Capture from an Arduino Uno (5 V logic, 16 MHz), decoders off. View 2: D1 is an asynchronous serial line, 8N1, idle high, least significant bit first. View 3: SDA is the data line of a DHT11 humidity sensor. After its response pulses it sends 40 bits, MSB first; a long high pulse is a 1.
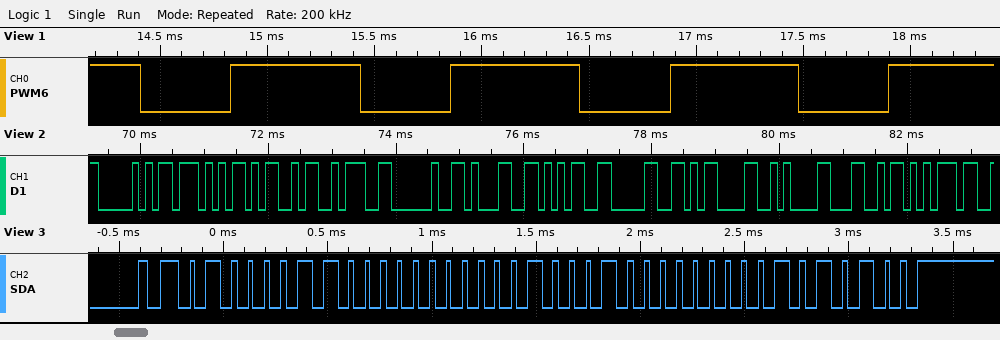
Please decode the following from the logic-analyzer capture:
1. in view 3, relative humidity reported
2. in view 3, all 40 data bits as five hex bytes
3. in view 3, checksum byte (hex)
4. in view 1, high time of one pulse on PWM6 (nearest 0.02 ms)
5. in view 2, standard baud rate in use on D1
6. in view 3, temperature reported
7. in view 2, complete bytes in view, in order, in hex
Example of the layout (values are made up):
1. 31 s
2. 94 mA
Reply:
1. 67 %
2. 43 00 11 00 54
3. 0x54
4. 0.60 ms
5. 9600 baud
6. 17.0 °C
7. 50 57 4D 3A 20 31 35 30 0D 0A 4C 75
